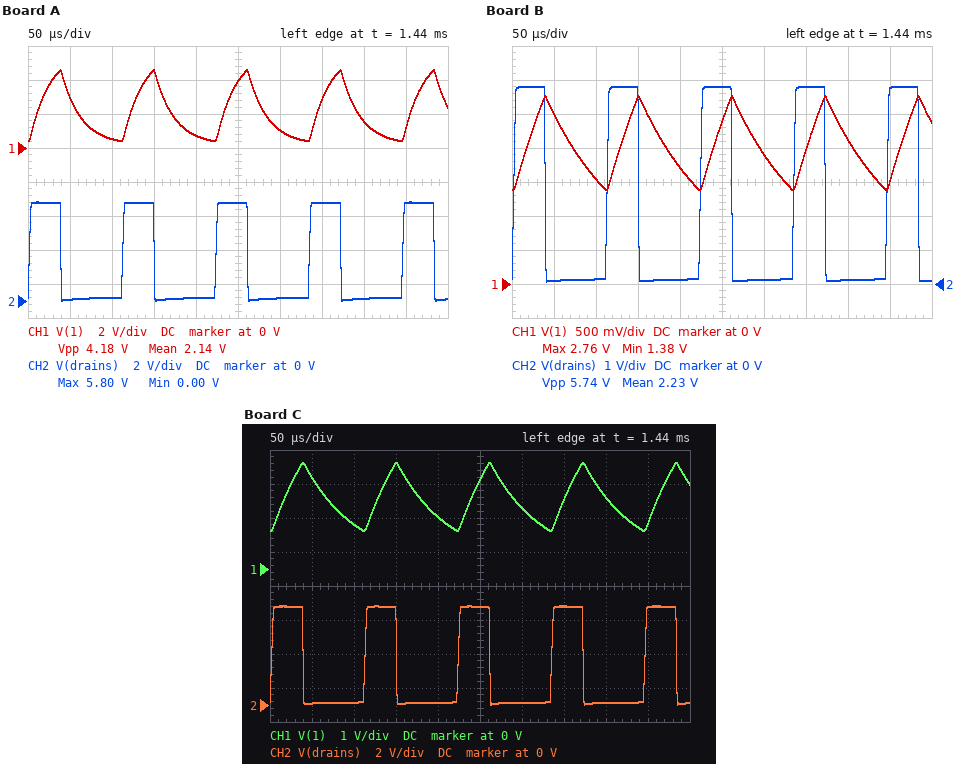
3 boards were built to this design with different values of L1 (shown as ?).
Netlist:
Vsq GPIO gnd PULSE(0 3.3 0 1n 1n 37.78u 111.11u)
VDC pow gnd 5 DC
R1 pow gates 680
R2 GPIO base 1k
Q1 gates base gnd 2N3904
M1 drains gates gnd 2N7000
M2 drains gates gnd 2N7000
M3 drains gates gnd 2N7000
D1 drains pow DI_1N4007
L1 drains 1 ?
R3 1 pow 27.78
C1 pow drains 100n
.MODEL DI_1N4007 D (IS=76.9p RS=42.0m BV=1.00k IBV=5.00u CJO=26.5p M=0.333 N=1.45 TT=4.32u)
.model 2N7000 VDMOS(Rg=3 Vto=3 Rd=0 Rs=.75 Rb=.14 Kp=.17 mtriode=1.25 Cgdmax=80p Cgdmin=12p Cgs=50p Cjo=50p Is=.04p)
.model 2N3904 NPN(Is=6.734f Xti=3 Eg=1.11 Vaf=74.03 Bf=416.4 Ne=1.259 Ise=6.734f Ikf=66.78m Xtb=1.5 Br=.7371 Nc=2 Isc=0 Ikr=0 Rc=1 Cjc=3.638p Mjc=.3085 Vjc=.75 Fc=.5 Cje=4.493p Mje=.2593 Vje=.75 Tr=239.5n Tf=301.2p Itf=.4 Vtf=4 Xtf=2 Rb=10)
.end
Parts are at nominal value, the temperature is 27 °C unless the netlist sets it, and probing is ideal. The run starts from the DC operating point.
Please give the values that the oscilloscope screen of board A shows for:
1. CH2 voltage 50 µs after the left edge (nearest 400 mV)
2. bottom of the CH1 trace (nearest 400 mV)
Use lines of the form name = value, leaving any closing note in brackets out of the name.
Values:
CH2 voltage 50 µs after the left edge = 0 V
bottom of the CH1 trace = 400 mV
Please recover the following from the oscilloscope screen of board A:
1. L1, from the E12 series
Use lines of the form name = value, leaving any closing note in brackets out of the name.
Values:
L1, from the E12 series = 680 µH
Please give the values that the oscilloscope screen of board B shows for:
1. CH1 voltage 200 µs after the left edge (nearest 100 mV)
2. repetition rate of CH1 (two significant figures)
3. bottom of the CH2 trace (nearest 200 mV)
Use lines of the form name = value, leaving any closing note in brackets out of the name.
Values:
CH1 voltage 200 µs after the left edge = 1.7 V
repetition rate of CH1 = 9.0 kHz
bottom of the CH2 trace = 0 V
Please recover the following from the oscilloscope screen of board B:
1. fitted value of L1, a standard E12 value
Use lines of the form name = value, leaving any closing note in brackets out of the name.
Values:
fitted value of L1, a standard E12 value = 2.7 mH
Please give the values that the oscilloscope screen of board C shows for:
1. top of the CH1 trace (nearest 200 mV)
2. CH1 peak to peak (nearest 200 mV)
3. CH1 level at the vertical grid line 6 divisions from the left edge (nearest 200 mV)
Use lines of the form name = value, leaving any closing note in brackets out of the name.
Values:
top of the CH1 trace = 3.2 V
CH1 peak to peak = 2.0 V
CH1 level at the vertical grid line 6 divisions from the left edge = 1.8 V
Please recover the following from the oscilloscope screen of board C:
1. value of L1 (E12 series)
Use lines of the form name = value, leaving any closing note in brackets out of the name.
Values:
value of L1 = 1.8 mH
